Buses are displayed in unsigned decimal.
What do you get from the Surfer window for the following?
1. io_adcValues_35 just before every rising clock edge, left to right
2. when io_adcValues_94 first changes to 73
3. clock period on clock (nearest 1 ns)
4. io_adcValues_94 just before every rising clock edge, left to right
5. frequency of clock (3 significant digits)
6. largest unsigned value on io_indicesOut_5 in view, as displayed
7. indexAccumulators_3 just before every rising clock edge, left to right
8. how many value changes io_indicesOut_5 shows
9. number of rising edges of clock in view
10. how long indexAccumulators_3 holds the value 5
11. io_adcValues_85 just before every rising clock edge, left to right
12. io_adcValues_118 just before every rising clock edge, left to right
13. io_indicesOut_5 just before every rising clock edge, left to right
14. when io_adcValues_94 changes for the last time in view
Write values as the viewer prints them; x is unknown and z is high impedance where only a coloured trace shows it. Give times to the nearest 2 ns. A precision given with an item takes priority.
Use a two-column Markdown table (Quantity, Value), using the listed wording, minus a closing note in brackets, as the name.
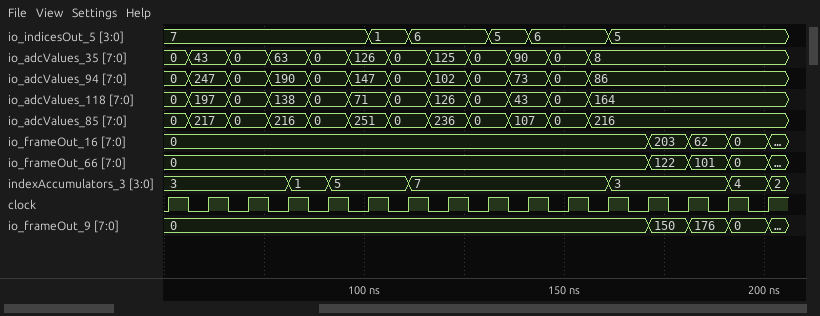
| Quantity | Value |
|---|---|
| io_adcValues_35 just before every rising clock edge, left to right | 0, 43, 0, 63, 0, 126, 0, 125, 0, 90, 0, 8, 8, 8, 8, 8 |
| when io_adcValues_94 first changes to 73 | 136 ns |
| clock period on clock | 10 ns |
| io_adcValues_94 just before every rising clock edge, left to right | 0, 247, 0, 190, 0, 147, 0, 102, 0, 73, 0, 86, 86, 86, 86, 86 |
| frequency of clock | 100 MHz |
| largest unsigned value on io_indicesOut_5 in view, as displayed | 7 |
| indexAccumulators_3 just before every rising clock edge, left to right | 3, 3, 3, 3, 1, 5, 5, 7, 7, 7, 7, 7, 3, 3, 3, 4 |
| how many value changes io_indicesOut_5 shows | 5 |
| number of rising edges of clock in view | 16 |
| how long indexAccumulators_3 holds the value 5 | 20 ns |
| io_adcValues_85 just before every rising clock edge, left to right | 0, 217, 0, 216, 0, 251, 0, 236, 0, 107, 0, 216, 216, 216, 216, 216 |
| io_adcValues_118 just before every rising clock edge, left to right | 0, 197, 0, 138, 0, 71, 0, 126, 0, 43, 0, 164, 164, 164, 164, 164 |
| io_indicesOut_5 just before every rising clock edge, left to right | 7, 7, 7, 7, 7, 7, 1, 6, 6, 5, 6, 6, 5, 5, 5, 5 |
| when io_adcValues_94 changes for the last time in view | 156 ns |
